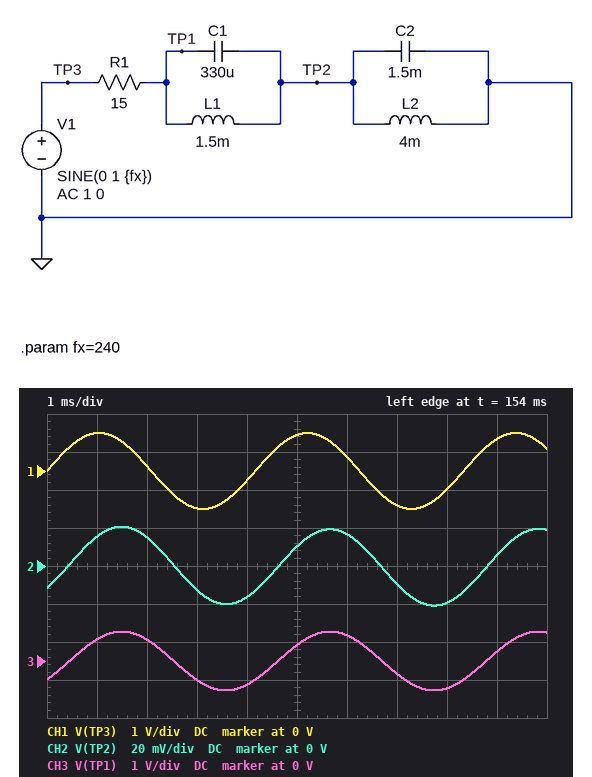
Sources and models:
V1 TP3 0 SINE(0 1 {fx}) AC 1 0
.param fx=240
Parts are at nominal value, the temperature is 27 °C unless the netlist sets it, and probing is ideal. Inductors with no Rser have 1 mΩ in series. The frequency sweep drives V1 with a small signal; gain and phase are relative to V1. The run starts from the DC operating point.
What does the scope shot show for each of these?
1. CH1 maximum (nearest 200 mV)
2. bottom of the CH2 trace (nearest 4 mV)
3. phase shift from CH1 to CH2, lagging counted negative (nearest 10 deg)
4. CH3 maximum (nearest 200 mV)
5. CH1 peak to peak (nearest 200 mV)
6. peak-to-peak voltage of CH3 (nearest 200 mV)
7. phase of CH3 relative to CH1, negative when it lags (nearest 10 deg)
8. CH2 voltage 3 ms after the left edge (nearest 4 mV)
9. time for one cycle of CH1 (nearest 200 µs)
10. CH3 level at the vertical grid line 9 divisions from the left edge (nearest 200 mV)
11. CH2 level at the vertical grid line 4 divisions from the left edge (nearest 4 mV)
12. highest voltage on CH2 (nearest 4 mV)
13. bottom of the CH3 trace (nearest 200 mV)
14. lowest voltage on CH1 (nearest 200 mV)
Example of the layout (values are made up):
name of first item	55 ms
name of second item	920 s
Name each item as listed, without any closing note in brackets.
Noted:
CH1 maximum	1.0 V
bottom of the CH2 trace	-20 mV
phase shift from CH1 to CH2, lagging counted negative	-40 deg
CH3 maximum	800 mV
CH1 peak to peak	2.0 V
peak-to-peak voltage of CH3	1.6 V
phase of CH3 relative to CH1, negative when it lags	-40 deg
CH2 voltage 3 ms after the left edge	-12 mV
time for one cycle of CH1	4.2 ms
CH3 level at the vertical grid line 9 divisions from the left edge	200 mV
CH2 level at the vertical grid line 4 divisions from the left edge	-16 mV
highest voltage on CH2	20 mV
bottom of the CH3 trace	-800 mV
lowest voltage on CH1	-1.0 V
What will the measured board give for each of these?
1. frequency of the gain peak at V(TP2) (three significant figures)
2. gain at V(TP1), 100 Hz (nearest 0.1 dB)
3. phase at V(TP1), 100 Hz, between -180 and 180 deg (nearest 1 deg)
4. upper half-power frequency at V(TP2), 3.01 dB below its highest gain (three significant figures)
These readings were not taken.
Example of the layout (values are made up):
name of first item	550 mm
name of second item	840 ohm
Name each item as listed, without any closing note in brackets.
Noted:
frequency of the gain peak at V(TP2)	65.1 Hz
gain at V(TP1), 100 Hz	-27.1 dB
phase at V(TP1), 100 Hz, between -180 and 180 deg	-87 deg
upper half-power frequency at V(TP2), 3.01 dB below its highest gain	68.8 Hz
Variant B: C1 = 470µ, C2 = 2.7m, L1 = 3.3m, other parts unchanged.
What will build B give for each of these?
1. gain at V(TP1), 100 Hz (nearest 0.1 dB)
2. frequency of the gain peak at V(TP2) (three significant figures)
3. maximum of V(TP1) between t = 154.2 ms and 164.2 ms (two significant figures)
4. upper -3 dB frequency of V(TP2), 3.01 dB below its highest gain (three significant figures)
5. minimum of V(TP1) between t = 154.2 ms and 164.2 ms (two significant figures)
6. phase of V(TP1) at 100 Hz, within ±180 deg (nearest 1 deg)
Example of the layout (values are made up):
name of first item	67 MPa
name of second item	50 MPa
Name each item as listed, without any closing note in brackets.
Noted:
gain at V(TP1), 100 Hz	-10.7 dB
frequency of the gain peak at V(TP2)	48.6 Hz
maximum of V(TP1) between t = 154.2 ms and 164.2 ms	150 mV
upper -3 dB frequency of V(TP2), 3.01 dB below its highest gain	50.6 Hz
minimum of V(TP1) between t = 154.2 ms and 164.2 ms	-150 mV
phase of V(TP1) at 100 Hz, within ±180 deg	73 deg
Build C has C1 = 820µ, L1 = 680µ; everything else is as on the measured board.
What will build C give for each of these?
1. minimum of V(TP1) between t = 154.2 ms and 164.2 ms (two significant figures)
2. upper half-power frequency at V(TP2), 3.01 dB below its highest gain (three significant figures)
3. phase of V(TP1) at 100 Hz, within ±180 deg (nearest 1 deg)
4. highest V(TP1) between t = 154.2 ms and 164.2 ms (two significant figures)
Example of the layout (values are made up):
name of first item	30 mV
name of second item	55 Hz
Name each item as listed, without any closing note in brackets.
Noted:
minimum of V(TP1) between t = 154.2 ms and 164.2 ms	-280 mV
upper half-power frequency at V(TP2), 3.01 dB below its highest gain	68.7 Hz
phase of V(TP1) at 100 Hz, within ±180 deg	-85 deg
highest V(TP1) between t = 154.2 ms and 164.2 ms	280 mV
